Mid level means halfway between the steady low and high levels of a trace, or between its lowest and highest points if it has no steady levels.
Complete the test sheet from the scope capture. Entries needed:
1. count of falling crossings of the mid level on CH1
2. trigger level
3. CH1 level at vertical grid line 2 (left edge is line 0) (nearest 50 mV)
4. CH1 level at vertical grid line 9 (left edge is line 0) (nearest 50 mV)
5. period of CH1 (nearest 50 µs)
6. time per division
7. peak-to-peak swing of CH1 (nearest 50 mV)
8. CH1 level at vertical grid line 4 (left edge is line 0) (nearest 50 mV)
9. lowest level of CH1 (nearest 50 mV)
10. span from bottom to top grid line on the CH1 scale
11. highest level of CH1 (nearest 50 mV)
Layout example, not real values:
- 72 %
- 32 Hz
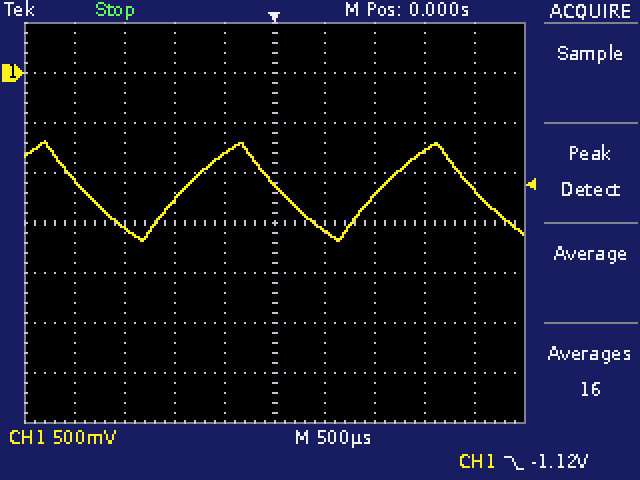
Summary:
- 3
- -1.12 V
- -1.55 V
- -1.15 V
- 1.95 ms
- 500 µs
- 1.00 V
- -800 mV
- -1.70 V
- 4 V
- -700 mV
